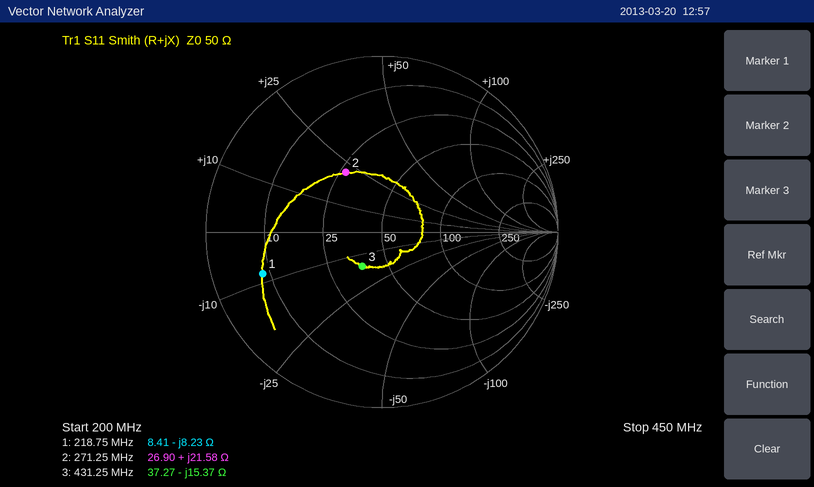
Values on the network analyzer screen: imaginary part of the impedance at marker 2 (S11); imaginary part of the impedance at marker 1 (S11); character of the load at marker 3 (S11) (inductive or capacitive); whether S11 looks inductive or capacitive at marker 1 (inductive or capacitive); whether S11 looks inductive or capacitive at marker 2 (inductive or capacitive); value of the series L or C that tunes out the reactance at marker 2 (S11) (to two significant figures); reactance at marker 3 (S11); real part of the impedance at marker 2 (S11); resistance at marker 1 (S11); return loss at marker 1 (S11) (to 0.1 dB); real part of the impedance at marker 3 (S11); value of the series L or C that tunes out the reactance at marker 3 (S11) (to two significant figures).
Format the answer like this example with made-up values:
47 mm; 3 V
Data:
+21.58 Ω; -8.23 Ω; capacitive; capacitive; inductive; 27 pF; -15.37 Ω; 26.90 Ω; 8.41 Ω; 2.9 dB; 37.27 Ω; 5.7 nH
